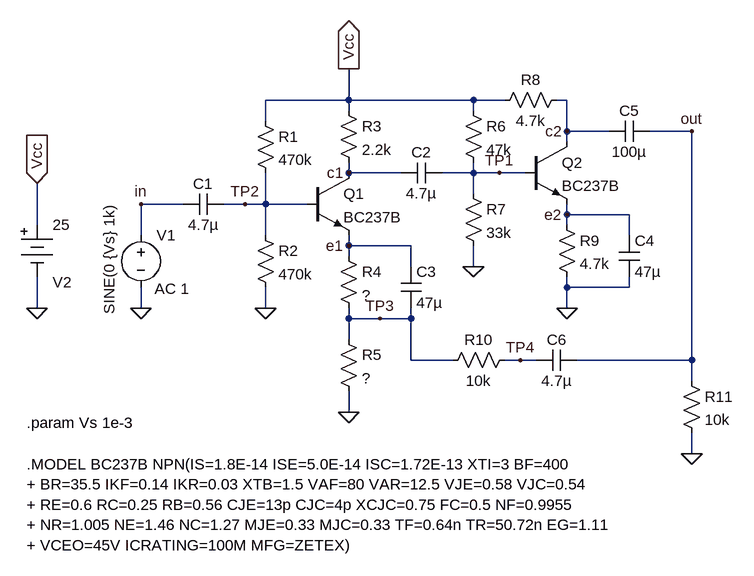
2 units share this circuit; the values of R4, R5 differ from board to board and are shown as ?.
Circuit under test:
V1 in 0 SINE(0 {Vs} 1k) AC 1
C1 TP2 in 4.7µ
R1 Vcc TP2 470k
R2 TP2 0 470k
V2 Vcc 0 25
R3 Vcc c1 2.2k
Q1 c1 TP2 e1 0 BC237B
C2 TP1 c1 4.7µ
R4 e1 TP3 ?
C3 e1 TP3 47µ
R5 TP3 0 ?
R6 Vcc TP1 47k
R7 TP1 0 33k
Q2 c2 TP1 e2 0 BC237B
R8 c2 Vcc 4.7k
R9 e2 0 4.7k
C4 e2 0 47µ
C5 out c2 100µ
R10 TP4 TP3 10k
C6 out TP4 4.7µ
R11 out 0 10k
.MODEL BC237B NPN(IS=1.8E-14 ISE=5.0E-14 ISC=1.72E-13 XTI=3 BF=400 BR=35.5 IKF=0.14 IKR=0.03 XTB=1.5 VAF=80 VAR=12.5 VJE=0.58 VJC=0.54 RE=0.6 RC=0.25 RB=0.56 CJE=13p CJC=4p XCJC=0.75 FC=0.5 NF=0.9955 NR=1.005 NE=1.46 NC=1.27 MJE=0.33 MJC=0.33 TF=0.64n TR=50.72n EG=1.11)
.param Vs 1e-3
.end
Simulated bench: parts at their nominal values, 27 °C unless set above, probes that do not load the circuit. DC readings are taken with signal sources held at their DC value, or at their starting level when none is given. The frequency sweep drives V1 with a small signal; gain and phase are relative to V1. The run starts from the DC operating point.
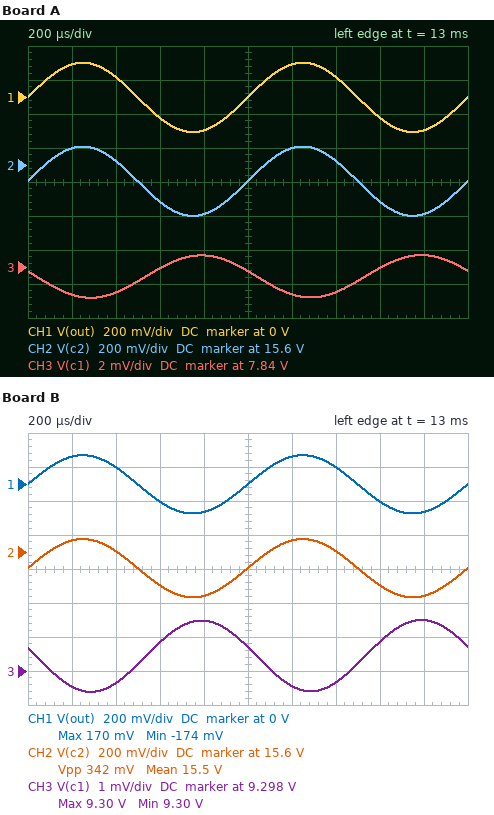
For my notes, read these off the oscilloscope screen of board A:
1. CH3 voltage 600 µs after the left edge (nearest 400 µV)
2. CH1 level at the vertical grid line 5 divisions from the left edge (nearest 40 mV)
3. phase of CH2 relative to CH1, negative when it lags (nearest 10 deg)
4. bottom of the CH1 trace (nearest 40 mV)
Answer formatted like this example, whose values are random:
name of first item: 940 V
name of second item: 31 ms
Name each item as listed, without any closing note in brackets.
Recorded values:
CH3 voltage 600 µs after the left edge: 7.8400 V
CH1 level at the vertical grid line 5 divisions from the left edge: 0 V
phase of CH2 relative to CH1, negative when it lags: 0 deg
bottom of the CH1 trace: -200 mV
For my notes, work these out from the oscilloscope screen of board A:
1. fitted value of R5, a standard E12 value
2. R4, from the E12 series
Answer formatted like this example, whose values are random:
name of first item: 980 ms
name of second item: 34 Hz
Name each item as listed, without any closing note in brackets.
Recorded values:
fitted value of R5, a standard E12 value: 47 Ω
R4, from the E12 series: 680 Ω
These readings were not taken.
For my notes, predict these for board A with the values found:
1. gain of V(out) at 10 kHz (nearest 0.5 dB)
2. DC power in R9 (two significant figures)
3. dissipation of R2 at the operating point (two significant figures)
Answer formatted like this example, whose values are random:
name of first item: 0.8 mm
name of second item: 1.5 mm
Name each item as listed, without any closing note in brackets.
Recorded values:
gain of V(out) at 10 kHz: 46.0 dB
DC power in R9: 19 mW
dissipation of R2 at the operating point: 87 µW
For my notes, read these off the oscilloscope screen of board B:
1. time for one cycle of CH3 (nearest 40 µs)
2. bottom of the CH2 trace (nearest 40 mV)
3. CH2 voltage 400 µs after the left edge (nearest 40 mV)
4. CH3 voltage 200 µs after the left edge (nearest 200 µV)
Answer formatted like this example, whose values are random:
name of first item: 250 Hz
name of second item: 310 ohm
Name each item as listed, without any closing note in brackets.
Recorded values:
time for one cycle of CH3: 1.00 ms
bottom of the CH2 trace: 15.32 V
CH2 voltage 400 µs after the left edge: 15.60 V
CH3 voltage 200 µs after the left edge: 9.2976 V
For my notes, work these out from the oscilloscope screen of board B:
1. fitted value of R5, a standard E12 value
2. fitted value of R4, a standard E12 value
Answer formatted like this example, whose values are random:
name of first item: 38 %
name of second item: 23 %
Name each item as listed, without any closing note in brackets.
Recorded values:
fitted value of R5, a standard E12 value: 56 Ω
fitted value of R4, a standard E12 value: 820 Ω
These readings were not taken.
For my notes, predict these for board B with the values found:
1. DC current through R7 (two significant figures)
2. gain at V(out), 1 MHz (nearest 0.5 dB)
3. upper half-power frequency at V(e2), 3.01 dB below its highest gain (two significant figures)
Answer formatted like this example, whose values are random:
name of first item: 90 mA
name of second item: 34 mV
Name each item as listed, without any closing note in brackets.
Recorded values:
DC current through R7: 310 µA
gain at V(out), 1 MHz: 44.5 dB
upper half-power frequency at V(e2), 3.01 dB below its highest gain: 28 Hz
